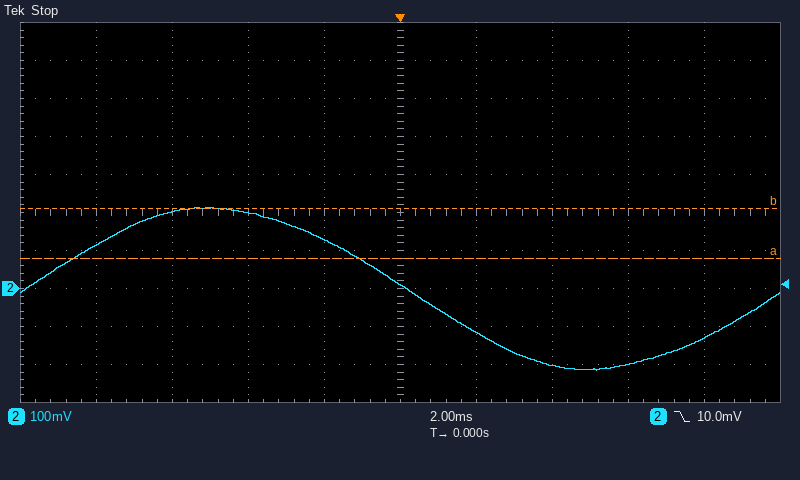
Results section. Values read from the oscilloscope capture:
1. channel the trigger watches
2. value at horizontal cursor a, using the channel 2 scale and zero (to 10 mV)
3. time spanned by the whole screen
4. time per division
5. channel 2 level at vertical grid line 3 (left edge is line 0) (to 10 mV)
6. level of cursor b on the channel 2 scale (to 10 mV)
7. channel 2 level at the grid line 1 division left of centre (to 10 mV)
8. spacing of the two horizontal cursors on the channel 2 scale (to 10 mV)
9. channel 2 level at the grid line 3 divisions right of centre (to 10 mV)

channel 2
80 mV
20 ms
2 ms
200 mV
210 mV
130 mV
130 mV
-200 mV
